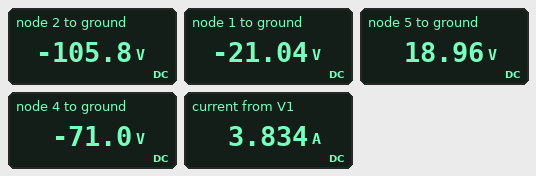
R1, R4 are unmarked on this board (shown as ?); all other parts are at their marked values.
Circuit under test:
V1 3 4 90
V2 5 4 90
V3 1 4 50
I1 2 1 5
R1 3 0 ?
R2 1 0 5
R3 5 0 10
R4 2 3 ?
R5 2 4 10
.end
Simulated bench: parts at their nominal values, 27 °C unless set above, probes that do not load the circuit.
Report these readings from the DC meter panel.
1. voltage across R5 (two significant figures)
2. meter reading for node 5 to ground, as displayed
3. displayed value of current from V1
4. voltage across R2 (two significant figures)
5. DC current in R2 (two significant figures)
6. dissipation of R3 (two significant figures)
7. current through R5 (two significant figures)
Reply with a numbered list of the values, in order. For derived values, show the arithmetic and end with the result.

1. -71 V - (-105.8 V) = 35 V
2. 18.96 V
3. 3.834 A
4. 0 V - (-21.04 V) = 21 V
5. (0 V - (-21.04 V)) / 5 Ω = 4.2 A
6. (18.96 V)^2 / 10 Ω = 36 W
7. (-71 V - (-105.8 V)) / 10 Ω = 3.5 A
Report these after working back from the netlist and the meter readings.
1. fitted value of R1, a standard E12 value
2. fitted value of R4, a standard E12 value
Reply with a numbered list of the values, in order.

1. 8.2 Ω
2. 82 Ω
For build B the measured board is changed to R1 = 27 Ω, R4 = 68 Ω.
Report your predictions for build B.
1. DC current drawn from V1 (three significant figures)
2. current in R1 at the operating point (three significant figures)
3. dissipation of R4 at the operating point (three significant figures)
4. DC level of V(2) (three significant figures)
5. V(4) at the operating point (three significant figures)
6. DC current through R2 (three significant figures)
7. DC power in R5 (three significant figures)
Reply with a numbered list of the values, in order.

1. 2.67 A
2. 879 mA
3. 219 W
4. -98.3 V
5. -66.3 V
6. 3.25 A
7. 103 W
